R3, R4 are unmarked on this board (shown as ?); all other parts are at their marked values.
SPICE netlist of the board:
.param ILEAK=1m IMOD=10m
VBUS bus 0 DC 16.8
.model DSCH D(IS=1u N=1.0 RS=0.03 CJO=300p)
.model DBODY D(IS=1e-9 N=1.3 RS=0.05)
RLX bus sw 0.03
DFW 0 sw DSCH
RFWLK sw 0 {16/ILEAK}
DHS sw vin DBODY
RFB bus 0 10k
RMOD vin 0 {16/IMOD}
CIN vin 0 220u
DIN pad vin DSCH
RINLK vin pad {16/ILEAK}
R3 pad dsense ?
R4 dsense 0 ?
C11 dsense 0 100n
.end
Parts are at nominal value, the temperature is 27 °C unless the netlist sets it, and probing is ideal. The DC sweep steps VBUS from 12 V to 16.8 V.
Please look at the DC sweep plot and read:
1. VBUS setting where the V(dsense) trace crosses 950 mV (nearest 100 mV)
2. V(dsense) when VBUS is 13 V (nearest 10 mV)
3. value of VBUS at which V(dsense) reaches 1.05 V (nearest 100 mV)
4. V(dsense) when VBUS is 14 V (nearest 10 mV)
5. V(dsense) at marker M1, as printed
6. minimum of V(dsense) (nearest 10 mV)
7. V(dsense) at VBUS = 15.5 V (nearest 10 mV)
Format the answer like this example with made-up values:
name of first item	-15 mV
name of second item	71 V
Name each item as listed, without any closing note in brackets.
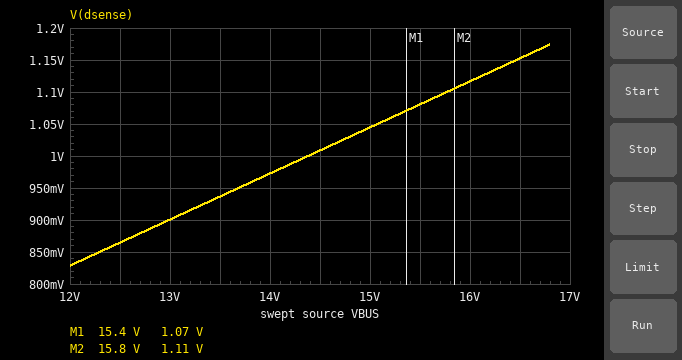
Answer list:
VBUS setting where the V(dsense) trace crosses 950 mV	13.7 V
V(dsense) when VBUS is 13 V	900 mV
value of VBUS at which V(dsense) reaches 1.05 V	15.1 V
V(dsense) when VBUS is 14 V	970 mV
V(dsense) at marker M1, as printed	1.07 V
minimum of V(dsense)	830 mV
V(dsense) at VBUS = 15.5 V	1.08 V
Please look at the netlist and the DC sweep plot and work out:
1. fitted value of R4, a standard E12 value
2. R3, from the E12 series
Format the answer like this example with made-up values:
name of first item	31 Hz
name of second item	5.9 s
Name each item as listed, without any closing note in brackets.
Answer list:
fitted value of R4, a standard E12 value	5.6 kΩ
R3, from the E12 series	56 kΩ
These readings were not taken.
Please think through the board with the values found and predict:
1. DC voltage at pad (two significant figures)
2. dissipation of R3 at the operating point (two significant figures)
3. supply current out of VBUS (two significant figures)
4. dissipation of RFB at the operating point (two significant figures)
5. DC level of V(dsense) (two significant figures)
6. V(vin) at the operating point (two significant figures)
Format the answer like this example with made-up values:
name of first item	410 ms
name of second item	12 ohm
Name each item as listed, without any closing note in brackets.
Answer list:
DC voltage at pad	13 V
dissipation of R3 at the operating point	2.5 mW
supply current out of VBUS	13 mA
dissipation of RFB at the operating point	28 mW
DC level of V(dsense)	1.2 V
V(vin) at the operating point	16 V
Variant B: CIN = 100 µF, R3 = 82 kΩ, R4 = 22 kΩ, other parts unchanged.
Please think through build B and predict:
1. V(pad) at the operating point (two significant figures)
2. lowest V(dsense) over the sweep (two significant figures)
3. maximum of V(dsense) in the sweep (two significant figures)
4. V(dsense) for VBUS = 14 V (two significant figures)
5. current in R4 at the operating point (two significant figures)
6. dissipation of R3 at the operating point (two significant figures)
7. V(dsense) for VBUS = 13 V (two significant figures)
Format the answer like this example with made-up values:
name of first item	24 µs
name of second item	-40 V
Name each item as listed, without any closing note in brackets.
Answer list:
V(pad) at the operating point	14 V
lowest V(dsense) over the sweep	2.1 V
maximum of V(dsense) in the sweep	3.0 V
V(dsense) for VBUS = 14 V	2.5 V
current in R4 at the operating point	140 µA
dissipation of R3 at the operating point	1.5 mW
V(dsense) for VBUS = 13 V	2.3 V
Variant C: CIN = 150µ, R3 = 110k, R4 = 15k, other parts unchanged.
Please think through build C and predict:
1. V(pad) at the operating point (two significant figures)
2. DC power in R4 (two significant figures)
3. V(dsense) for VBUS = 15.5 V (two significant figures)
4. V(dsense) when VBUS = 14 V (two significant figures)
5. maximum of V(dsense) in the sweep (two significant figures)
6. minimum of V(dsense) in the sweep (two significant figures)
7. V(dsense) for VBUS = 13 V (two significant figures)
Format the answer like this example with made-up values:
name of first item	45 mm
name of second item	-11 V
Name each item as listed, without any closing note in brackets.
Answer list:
V(pad) at the operating point	14 V
DC power in R4	200 µW
V(dsense) for VBUS = 15.5 V	1.6 V
V(dsense) when VBUS = 14 V	1.4 V
maximum of V(dsense) in the sweep	1.7 V
minimum of V(dsense) in the sweep	1.2 V
V(dsense) for VBUS = 13 V	1.3 V
